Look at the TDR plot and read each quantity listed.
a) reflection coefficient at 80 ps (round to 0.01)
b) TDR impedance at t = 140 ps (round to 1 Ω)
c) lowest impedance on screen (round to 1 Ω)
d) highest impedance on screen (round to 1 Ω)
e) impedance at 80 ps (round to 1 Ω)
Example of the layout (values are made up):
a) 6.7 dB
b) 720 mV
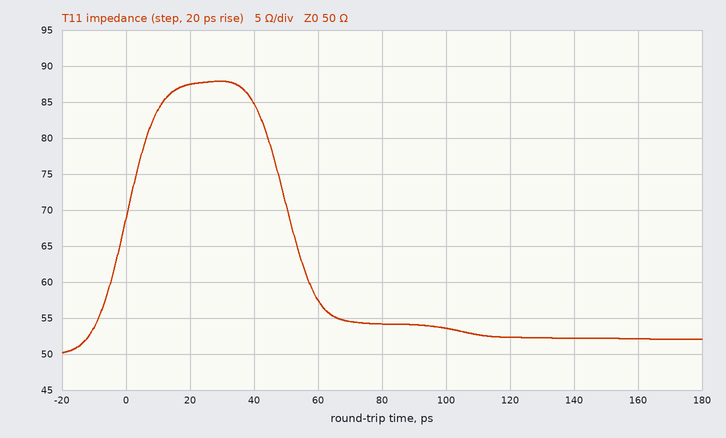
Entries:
a) +0.04
b) 52 Ω
c) 50 Ω
d) 88 Ω
e) 54 Ω
